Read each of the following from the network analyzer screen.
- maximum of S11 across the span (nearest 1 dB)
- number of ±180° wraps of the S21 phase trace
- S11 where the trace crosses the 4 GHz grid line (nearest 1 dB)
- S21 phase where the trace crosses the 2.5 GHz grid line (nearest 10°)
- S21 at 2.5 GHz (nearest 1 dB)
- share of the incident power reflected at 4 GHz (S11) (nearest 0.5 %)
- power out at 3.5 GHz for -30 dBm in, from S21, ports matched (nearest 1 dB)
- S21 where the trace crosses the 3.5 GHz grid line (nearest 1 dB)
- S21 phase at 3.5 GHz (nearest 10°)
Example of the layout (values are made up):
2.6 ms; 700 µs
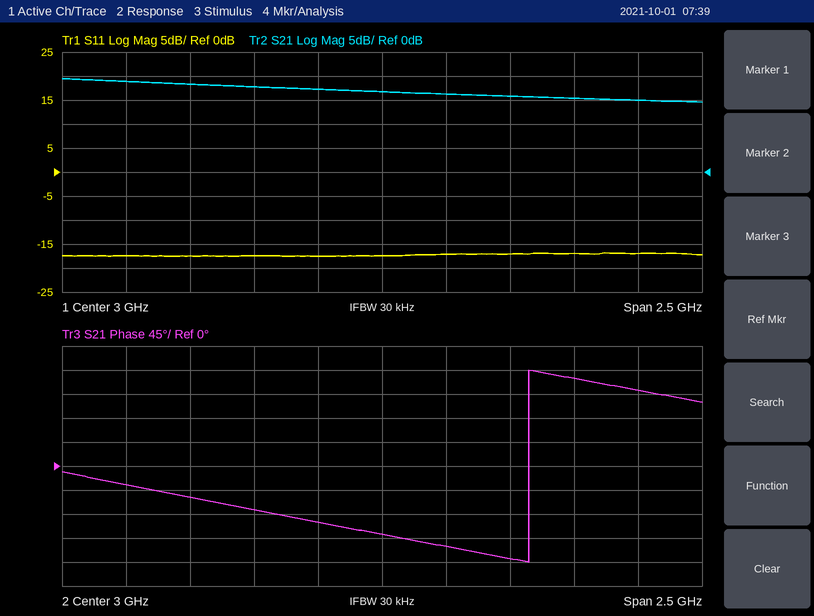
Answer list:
-17 dB; 1; -17 dB; -80°; 18 dB; 2.0 %; -14 dBm; 16 dB; -170°
